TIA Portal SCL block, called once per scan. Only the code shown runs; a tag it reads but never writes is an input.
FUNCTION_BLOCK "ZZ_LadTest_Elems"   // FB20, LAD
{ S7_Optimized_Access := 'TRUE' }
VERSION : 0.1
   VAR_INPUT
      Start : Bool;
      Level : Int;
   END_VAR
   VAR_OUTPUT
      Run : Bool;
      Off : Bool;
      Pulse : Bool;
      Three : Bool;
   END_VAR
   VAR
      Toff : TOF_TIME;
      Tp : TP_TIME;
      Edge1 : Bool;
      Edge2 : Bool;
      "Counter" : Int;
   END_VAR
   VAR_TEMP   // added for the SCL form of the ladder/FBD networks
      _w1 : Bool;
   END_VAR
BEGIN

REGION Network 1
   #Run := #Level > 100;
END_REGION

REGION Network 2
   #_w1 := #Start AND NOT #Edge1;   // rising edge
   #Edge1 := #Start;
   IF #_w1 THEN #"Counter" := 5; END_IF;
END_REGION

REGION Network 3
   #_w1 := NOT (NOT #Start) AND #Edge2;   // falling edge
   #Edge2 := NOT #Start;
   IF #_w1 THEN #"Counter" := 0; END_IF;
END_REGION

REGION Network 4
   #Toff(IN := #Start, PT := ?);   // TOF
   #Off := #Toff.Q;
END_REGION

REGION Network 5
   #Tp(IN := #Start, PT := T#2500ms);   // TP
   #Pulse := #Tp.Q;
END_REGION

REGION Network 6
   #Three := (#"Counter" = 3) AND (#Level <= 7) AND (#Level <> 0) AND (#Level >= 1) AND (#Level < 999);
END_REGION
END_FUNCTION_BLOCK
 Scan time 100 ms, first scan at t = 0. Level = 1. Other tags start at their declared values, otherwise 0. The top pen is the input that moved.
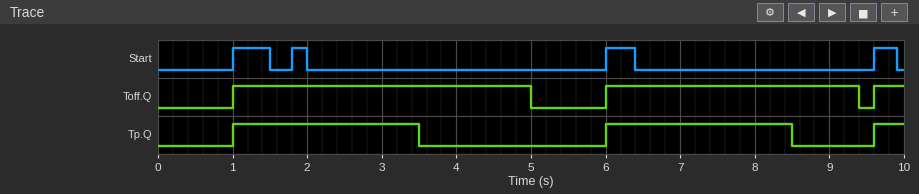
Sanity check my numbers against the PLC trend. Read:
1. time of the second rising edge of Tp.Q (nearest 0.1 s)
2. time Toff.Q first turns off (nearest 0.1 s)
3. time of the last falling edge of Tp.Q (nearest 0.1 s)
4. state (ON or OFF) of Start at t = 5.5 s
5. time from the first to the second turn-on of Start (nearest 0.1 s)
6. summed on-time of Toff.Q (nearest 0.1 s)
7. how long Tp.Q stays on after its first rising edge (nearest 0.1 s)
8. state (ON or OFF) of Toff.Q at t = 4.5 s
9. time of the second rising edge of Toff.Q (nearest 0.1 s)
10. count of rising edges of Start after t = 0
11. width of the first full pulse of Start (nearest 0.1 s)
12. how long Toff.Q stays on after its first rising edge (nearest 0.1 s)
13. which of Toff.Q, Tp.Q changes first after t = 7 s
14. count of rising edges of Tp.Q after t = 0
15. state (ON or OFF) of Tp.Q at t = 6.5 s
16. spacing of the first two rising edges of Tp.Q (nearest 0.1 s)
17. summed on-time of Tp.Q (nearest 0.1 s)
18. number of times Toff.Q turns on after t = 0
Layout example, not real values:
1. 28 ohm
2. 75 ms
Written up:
1. 6.0 s
2. 5.0 s
3. 8.5 s
4. OFF
5. 0.8 s
6. 7.8 s
7. 2.5 s
8. ON
9. 6.0 s
10. 4
11. 0.5 s
12. 4.0 s
13. Tp.Q
14. 3
15. ON
16. 5.0 s
17. 5.4 s
18. 3
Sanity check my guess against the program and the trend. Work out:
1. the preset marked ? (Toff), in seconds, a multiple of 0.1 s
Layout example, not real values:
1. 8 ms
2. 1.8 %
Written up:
1. 3.0 s
